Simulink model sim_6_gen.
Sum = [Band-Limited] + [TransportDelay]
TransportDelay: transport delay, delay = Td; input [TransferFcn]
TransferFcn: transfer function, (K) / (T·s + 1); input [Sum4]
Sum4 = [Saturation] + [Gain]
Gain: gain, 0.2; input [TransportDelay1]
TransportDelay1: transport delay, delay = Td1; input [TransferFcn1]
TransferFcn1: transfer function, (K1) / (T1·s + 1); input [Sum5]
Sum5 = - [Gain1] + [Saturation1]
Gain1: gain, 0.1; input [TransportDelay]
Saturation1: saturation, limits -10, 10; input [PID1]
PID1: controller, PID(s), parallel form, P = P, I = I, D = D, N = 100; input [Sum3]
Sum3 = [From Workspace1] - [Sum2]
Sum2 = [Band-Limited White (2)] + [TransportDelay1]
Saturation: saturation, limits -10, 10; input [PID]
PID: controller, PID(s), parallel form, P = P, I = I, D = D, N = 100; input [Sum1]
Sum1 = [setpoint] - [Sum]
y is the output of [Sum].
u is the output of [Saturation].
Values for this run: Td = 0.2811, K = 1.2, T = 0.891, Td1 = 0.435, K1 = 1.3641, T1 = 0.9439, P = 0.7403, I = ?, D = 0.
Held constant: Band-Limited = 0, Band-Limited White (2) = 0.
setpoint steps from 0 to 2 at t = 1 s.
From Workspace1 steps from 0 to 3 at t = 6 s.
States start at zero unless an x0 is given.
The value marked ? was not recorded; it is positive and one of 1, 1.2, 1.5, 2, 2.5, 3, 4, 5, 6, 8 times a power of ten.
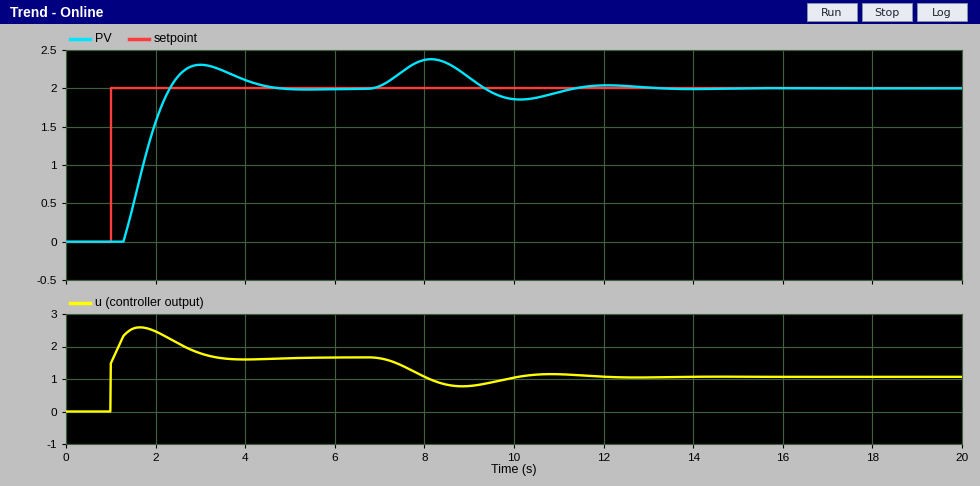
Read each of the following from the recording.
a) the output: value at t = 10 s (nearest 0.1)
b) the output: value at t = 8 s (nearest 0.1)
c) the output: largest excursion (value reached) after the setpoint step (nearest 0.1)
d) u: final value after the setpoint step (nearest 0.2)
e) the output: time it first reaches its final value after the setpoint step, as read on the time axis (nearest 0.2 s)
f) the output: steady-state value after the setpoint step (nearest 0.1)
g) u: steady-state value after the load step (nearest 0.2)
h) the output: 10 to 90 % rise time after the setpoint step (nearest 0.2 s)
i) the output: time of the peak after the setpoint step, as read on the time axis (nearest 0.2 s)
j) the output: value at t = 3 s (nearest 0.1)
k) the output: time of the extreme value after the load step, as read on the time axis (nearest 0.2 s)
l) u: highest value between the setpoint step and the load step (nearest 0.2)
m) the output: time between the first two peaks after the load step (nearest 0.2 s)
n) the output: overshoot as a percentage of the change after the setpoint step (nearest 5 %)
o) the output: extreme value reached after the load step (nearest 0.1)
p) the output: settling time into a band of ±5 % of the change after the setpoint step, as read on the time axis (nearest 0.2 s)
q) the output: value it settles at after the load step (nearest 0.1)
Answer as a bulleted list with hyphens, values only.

- 1.9
- 2.4
- 2.3
- 1.6
- 2.4 s
- 2.0
- 1.0
- 0.8 s
- 3.0 s
- 2.3
- 8.2 s
- 2.6
- 4.0 s
- 15 %
- 2.4
- 4.0 s
- 2.0
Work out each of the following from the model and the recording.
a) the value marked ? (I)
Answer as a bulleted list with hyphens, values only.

- 1.5
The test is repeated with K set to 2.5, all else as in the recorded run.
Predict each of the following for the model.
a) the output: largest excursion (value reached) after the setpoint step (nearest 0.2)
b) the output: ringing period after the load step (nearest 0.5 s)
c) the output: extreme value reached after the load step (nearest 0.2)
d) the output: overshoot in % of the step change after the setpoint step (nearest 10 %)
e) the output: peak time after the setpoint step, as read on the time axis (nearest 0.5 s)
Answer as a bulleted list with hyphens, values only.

- 2.8
- 3.5 s
- 2.6
- 40 %
- 2.0 s
